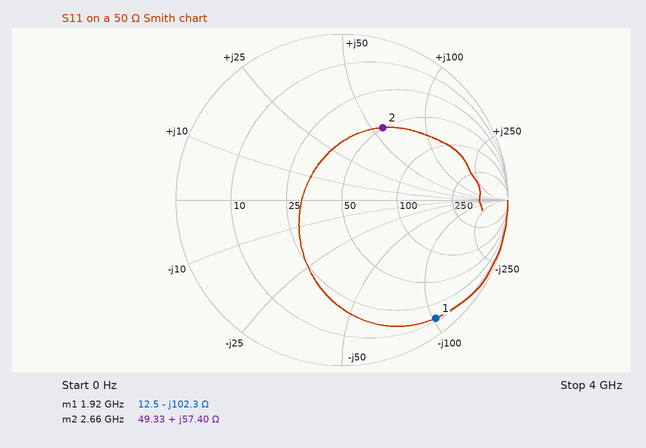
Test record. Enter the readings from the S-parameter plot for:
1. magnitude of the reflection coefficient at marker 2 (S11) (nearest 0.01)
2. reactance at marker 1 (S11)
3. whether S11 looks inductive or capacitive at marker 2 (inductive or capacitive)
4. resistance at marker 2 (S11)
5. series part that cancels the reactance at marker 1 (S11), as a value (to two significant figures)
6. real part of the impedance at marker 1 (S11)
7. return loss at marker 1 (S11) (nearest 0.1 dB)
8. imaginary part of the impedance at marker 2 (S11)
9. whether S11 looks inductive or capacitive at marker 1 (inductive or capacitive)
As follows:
0.50
-102.3 Ω
inductive
49.33 Ω
8.5 nH
12.5 Ω
0.8 dB
+57.40 Ω
capacitive
